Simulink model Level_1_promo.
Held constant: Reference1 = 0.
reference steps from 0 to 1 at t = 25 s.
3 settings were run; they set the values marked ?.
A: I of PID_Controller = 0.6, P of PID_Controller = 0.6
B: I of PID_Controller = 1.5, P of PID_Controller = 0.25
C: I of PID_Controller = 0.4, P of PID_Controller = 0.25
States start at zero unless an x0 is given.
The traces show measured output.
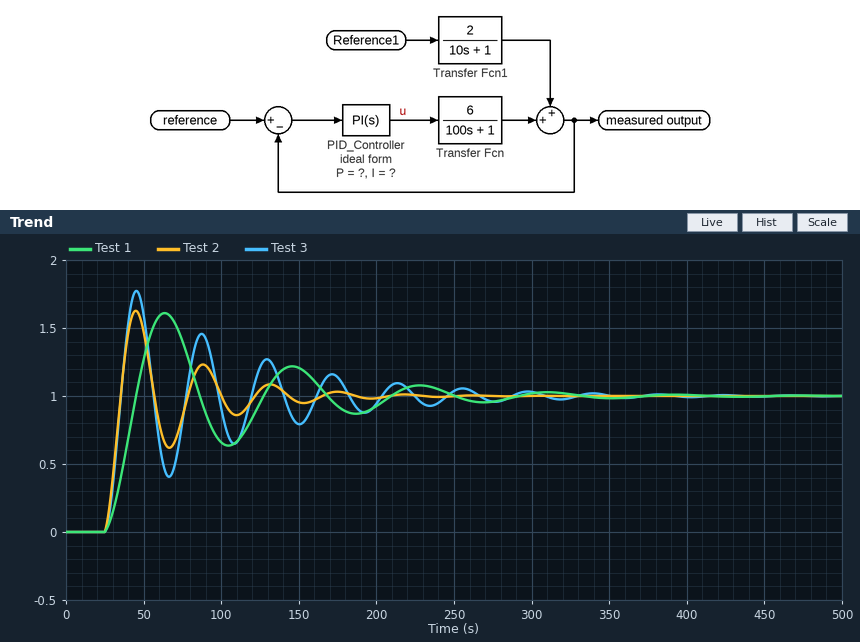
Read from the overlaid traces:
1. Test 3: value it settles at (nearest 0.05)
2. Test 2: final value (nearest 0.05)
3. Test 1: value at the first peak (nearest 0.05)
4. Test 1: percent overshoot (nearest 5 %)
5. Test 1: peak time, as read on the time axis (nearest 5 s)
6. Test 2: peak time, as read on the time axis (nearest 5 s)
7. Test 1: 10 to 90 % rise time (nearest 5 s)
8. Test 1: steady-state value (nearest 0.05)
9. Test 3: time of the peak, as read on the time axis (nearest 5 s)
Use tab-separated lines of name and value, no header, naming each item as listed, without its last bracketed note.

Test 3: value it settles at	1.00
Test 2: final value	1.00
Test 1: value at the first peak	1.60
Test 1: percent overshoot	60 %
Test 1: peak time, as read on the time axis	65 s
Test 2: peak time, as read on the time axis	45 s
Test 1: 10 to 90 % rise time	15 s
Test 1: steady-state value	1.00
Test 3: time of the peak, as read on the time axis	45 s
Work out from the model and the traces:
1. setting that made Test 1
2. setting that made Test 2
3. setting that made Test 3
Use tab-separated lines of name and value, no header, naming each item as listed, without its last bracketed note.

setting that made Test 1	C
setting that made Test 2	A
setting that made Test 3	B
